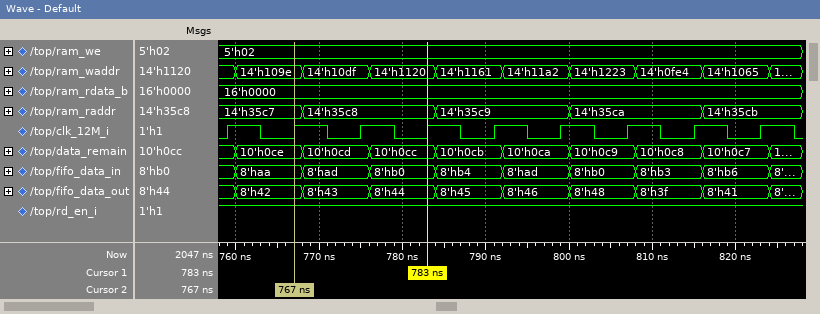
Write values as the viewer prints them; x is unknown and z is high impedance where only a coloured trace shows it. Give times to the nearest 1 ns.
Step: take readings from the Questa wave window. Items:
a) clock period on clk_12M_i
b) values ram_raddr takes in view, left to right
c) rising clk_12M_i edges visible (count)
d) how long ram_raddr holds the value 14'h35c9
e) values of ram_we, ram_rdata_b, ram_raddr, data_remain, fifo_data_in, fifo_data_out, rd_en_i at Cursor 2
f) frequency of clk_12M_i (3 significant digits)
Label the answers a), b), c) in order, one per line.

a) 8 ns
b) 14'h35c7, 14'h35c8, 14'h35c9, 14'h35ca, 14'h35cb
c) 9
d) 16 ns
e) ram_we=5'h02, ram_rdata_b=16'h0000, ram_raddr=14'h35c7, data_remain=10'h0ce, fifo_data_in=8'haa, fifo_data_out=8'h42, rd_en_i=1
f) 125 MHz
